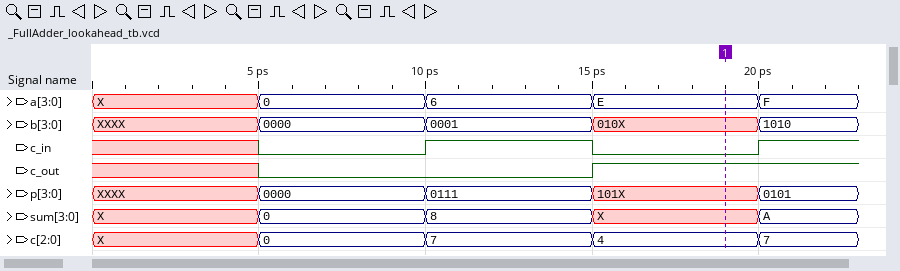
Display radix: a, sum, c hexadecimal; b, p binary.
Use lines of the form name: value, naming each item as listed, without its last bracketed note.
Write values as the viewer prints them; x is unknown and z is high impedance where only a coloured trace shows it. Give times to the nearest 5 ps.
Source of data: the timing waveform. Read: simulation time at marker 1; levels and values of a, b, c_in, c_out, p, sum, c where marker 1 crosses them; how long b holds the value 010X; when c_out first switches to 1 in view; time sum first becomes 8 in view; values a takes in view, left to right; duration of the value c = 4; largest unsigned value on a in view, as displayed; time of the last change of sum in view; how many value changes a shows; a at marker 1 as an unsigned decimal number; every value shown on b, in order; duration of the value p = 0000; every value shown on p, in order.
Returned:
simulation time at marker 1: 20 ps
levels and values of a, b, c_in, c_out, p, sum, c where marker 1 crosses them: a=E, b=010X, c_in=0, c_out=1, p=101X, sum=X, c=4
how long b holds the value 010X: 5 ps
when c_out first switches to 1 in view: 15 ps
time sum first becomes 8 in view: 10 ps
values a takes in view, left to right: X, 0, 6, E, F
duration of the value c = 4: 5 ps
largest unsigned value on a in view, as displayed: F
time of the last change of sum in view: 20 ps
how many value changes a shows: 4
a at marker 1 as an unsigned decimal number: 14
every value shown on b, in order: XXXX, 0000, 0001, 010X, 1010
duration of the value p = 0000: 5 ps
every value shown on p, in order: XXXX, 0000, 0111, 101X, 0101
